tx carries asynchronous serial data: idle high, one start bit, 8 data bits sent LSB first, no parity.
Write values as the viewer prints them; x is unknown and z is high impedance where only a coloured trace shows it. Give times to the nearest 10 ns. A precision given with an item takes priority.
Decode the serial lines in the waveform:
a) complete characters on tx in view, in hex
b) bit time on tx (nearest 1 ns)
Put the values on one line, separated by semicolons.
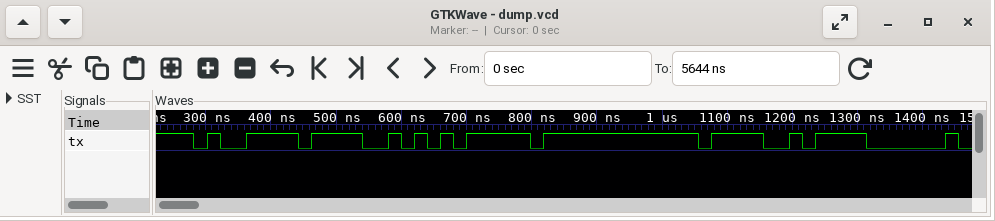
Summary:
79, AA, FF, 4F; 20 ns
